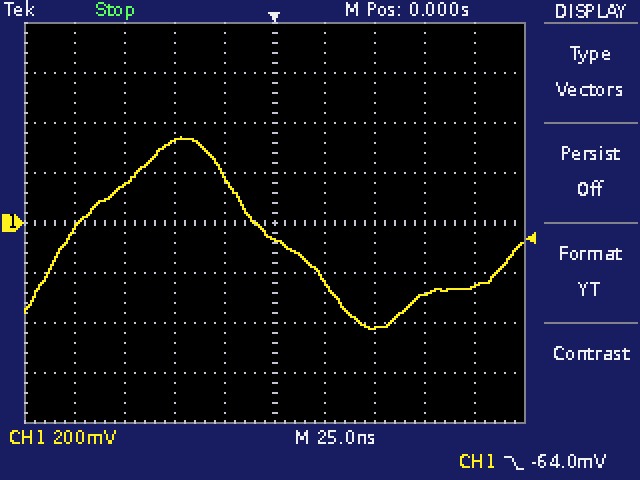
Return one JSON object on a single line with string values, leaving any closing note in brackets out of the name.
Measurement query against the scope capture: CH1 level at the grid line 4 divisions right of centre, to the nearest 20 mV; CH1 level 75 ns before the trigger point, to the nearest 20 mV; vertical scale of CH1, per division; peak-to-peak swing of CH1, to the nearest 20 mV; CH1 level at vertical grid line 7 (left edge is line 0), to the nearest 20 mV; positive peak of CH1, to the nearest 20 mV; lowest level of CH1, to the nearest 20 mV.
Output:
{"CH1 level at the grid line 4 divisions right of centre, to the nearest 20 mV": "-260 mV", "CH1 level 75 ns before the trigger point, to the nearest 20 mV": "160 mV", "vertical scale of CH1, per division": "200 mV", "peak-to-peak swing of CH1, to the nearest 20 mV": "760 mV", "CH1 level at vertical grid line 7 (left edge is line 0), to the nearest 20 mV": "-420 mV", "positive peak of CH1, to the nearest 20 mV": "340 mV", "lowest level of CH1, to the nearest 20 mV": "-420 mV"}
